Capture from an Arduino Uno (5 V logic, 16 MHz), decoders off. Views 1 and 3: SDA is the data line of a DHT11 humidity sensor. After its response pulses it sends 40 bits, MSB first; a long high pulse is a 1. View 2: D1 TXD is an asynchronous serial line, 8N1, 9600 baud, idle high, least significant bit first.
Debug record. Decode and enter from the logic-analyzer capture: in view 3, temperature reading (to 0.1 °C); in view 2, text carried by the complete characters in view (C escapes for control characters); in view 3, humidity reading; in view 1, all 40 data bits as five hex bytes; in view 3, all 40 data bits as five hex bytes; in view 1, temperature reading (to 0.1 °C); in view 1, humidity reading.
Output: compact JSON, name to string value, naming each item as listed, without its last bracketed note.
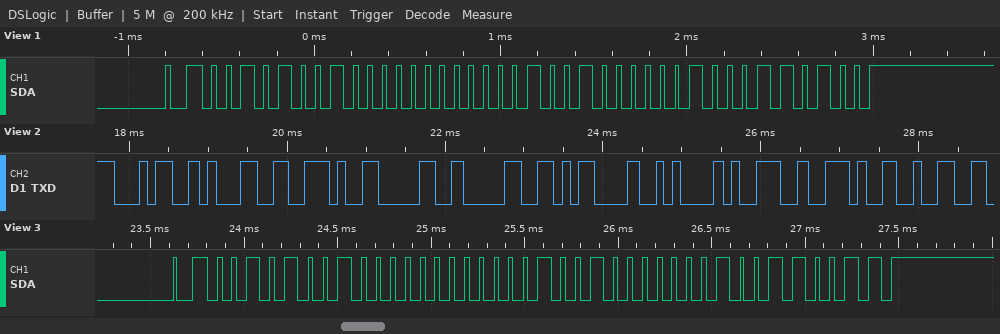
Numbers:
{"in view 3, temperature reading": "9.1 °C", "in view 2, text carried by the complete characters in view": "\"41.00\\r\\n9.2\"", "in view 3, humidity reading": "41 %", "in view 1, all 40 data bits as five hex bytes": "29 00 09 02 34", "in view 3, all 40 data bits as five hex bytes": "29 00 09 01 33", "in view 1, temperature reading": "9.2 °C", "in view 1, humidity reading": "41 %"}
